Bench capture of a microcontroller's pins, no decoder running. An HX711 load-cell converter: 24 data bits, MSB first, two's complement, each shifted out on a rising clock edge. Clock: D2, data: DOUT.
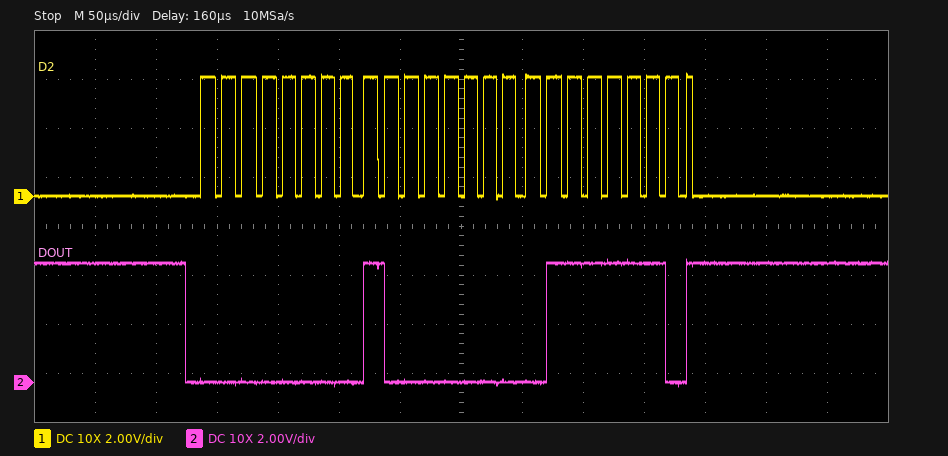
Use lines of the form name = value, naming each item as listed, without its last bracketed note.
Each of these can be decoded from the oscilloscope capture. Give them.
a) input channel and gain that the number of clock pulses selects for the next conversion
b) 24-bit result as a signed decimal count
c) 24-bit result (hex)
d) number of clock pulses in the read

input channel and gain that the number of clock pulses selects for the next conversion = channel A, gain 128
24-bit result as a signed decimal count = 32894
24-bit result = 0x00807E
number of clock pulses in the read = 25
